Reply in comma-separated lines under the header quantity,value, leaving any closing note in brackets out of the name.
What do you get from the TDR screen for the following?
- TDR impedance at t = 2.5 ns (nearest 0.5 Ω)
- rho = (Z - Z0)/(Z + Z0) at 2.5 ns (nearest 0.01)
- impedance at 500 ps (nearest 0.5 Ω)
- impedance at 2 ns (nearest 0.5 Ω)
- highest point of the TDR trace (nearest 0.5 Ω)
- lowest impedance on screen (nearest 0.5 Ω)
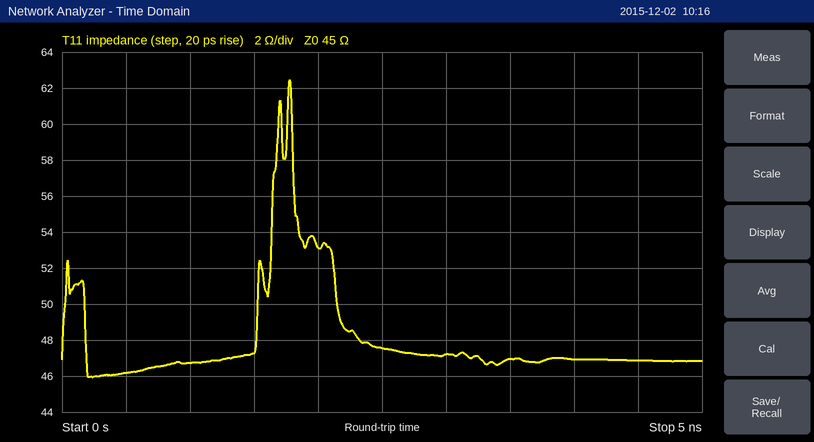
quantity,value
TDR impedance at t = 2.5 ns,47.5 Ω
rho = (Z - Z0)/(Z + Z0) at 2.5 ns,+0.03
impedance at 500 ps,46.0 Ω
impedance at 2 ns,53.0 Ω
highest point of the TDR trace,62.5 Ω
lowest impedance on screen,46.0 Ω
